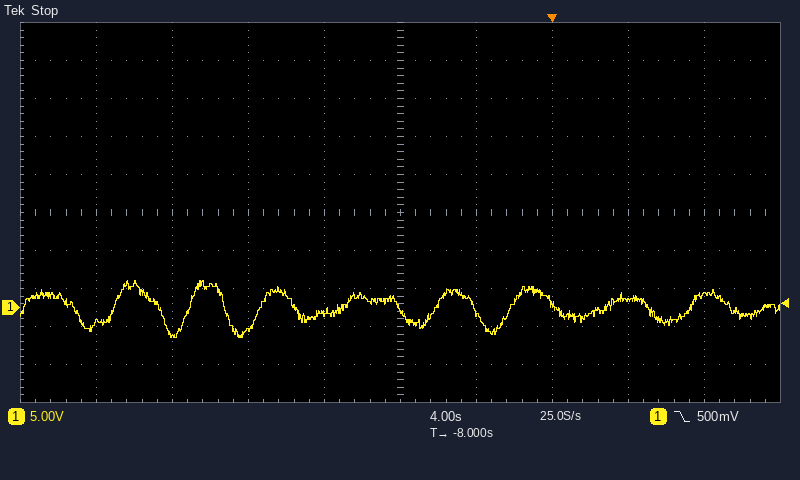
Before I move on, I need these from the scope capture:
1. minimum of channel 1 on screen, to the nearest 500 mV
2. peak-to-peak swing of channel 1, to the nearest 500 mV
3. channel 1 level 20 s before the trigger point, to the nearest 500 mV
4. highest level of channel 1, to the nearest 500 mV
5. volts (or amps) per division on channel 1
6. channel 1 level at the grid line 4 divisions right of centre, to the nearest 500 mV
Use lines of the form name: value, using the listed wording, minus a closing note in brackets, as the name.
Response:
minimum of channel 1 on screen, to the nearest 500 mV: -4.0 V
peak-to-peak swing of channel 1, to the nearest 500 mV: 7.5 V
channel 1 level 20 s before the trigger point, to the nearest 500 mV: -3.5 V
highest level of channel 1, to the nearest 500 mV: 3.5 V
volts (or amps) per division on channel 1: 5 V
channel 1 level at the grid line 4 divisions right of centre, to the nearest 500 mV: 1.5 V
